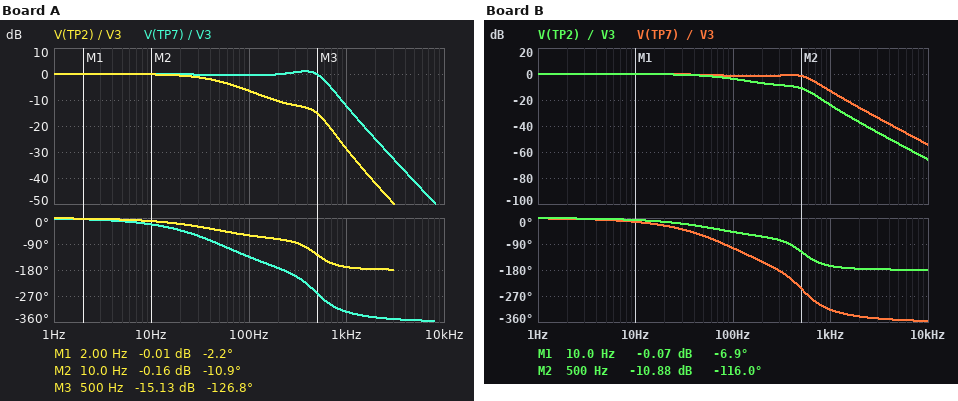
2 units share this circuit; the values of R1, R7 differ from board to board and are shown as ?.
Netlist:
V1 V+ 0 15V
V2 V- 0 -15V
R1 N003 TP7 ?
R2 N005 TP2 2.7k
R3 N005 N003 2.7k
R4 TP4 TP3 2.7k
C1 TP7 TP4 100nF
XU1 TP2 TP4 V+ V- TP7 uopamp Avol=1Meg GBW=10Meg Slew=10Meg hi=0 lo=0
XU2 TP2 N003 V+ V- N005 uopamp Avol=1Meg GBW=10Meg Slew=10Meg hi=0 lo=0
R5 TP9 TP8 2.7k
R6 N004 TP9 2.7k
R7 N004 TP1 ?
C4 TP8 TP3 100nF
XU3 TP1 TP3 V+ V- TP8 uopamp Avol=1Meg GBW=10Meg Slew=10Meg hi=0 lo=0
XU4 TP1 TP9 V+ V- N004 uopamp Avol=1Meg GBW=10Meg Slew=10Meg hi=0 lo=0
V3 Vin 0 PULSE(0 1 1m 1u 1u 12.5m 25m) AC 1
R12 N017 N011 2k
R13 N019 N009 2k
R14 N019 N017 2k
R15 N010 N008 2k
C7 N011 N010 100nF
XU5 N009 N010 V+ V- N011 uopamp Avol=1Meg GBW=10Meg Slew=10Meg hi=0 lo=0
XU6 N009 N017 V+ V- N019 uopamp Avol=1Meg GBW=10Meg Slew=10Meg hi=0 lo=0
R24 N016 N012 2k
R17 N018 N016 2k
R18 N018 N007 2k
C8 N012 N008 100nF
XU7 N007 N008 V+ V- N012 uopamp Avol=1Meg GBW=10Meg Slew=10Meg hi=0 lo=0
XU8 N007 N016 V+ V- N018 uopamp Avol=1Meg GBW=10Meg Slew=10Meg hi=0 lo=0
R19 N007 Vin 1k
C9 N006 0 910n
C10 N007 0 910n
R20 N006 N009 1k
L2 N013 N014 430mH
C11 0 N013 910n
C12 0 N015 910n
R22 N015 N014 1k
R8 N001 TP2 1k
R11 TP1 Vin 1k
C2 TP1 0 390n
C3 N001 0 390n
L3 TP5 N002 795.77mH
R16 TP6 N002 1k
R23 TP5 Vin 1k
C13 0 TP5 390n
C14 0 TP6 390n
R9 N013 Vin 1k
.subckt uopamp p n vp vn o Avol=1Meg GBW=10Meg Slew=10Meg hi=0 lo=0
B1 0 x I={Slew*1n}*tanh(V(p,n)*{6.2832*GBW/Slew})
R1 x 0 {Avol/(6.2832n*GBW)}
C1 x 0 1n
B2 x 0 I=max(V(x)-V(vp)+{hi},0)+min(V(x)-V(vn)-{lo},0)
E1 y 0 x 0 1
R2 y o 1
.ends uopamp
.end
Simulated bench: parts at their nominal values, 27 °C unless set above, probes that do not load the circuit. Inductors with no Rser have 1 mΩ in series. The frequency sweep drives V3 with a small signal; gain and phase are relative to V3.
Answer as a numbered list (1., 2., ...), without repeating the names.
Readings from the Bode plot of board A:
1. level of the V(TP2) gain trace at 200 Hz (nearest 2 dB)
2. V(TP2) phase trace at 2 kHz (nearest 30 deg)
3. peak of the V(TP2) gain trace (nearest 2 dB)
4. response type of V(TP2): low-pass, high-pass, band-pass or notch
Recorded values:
1. -10 dB
2. -180 deg
3. 0 dB
4. low-pass
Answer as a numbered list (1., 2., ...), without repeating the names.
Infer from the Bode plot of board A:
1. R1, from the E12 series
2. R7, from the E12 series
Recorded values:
1. 8.2 kΩ
2. 1.2 kΩ
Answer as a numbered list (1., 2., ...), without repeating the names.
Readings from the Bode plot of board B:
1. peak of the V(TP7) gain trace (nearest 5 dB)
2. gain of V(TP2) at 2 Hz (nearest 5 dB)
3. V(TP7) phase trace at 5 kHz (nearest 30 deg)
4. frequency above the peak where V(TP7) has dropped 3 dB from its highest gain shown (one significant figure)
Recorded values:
1. 0 dB
2. 0 dB
3. -360 deg
4. 600 Hz
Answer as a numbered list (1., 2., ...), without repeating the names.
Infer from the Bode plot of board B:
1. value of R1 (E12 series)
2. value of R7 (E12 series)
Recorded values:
1. 4.7 kΩ
2. 1.2 kΩ
